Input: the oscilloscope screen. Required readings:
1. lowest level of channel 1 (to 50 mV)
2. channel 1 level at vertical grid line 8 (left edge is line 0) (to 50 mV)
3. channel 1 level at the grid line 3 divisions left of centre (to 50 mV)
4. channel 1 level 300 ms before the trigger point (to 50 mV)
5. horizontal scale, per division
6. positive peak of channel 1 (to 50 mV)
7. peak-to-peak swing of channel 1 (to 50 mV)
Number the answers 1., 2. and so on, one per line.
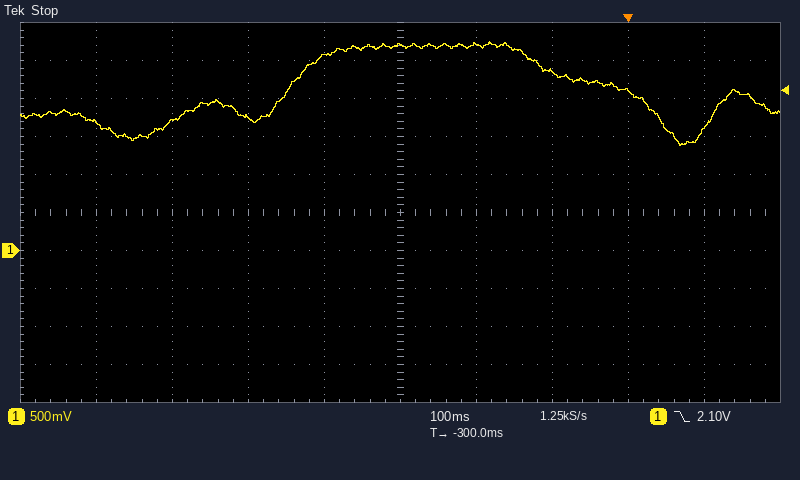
1. 1.40 V
2. 2.10 V
3. 1.70 V
4. 2.70 V
5. 100 ms
6. 2.75 V
7. 1.35 V
